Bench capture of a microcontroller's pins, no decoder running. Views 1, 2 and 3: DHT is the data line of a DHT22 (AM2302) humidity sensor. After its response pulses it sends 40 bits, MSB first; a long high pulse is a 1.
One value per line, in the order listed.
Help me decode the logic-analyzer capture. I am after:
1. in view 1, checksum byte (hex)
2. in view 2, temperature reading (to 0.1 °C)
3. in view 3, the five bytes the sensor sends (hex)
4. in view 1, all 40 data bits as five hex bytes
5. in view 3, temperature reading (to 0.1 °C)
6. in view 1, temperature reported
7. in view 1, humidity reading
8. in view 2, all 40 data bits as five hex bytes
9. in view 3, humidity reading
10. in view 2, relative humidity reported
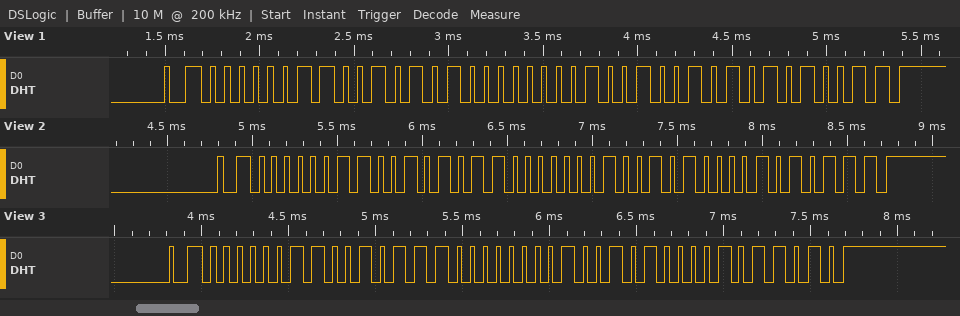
0x53
29.6 °C
03 2E 01 28 5A
03 2A 01 25 53
29.6 °C
29.3 °C
81.0 %
03 2B 01 28 57
81.4 %
81.1 %
